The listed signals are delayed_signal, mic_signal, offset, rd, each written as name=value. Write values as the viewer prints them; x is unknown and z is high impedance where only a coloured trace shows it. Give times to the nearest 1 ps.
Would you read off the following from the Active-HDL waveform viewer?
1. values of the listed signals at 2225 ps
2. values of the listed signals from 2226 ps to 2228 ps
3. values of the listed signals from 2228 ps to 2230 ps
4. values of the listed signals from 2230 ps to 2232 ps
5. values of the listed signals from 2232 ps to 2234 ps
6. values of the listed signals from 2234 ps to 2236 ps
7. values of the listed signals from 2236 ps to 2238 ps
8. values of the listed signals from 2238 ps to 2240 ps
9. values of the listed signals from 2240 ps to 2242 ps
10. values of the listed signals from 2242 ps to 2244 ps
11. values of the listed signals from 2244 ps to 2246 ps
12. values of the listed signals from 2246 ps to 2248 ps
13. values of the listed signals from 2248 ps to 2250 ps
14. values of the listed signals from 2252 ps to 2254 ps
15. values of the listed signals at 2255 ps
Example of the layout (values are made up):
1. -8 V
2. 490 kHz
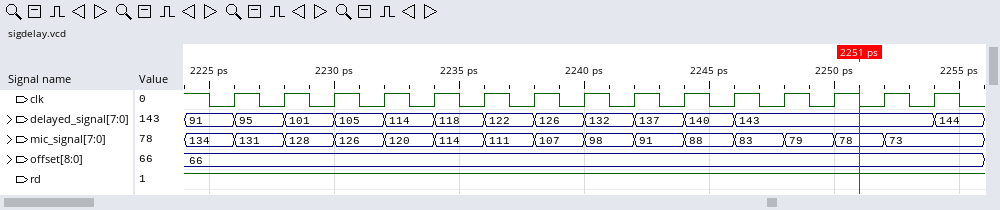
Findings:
1. delayed_signal=91, mic_signal=134, offset=66, rd=1
2. delayed_signal=95, mic_signal=131, offset=66, rd=1
3. delayed_signal=101, mic_signal=128, offset=66, rd=1
4. delayed_signal=105, mic_signal=126, offset=66, rd=1
5. delayed_signal=114, mic_signal=120, offset=66, rd=1
6. delayed_signal=118, mic_signal=114, offset=66, rd=1
7. delayed_signal=122, mic_signal=111, offset=66, rd=1
8. delayed_signal=126, mic_signal=107, offset=66, rd=1
9. delayed_signal=132, mic_signal=98, offset=66, rd=1
10. delayed_signal=137, mic_signal=91, offset=66, rd=1
11. delayed_signal=140, mic_signal=88, offset=66, rd=1
12. delayed_signal=143, mic_signal=83, offset=66, rd=1
13. delayed_signal=143, mic_signal=79, offset=66, rd=1
14. delayed_signal=143, mic_signal=73, offset=66, rd=1
15. delayed_signal=144, mic_signal=73, offset=66, rd=1
